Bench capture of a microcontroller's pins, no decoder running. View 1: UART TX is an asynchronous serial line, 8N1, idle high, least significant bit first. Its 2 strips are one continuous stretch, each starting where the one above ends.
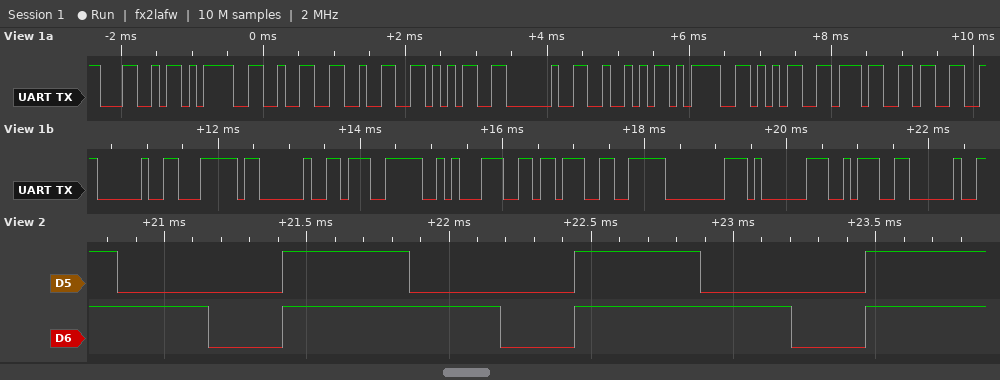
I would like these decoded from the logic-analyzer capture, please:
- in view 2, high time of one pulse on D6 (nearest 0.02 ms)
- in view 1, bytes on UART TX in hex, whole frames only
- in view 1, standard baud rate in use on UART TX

0.76 ms
4C 3D 32 32 35 20 52 3D 35 37 33 20 7C 20 E7 8A B6 E6 80 81 3A 20
9600 baud
